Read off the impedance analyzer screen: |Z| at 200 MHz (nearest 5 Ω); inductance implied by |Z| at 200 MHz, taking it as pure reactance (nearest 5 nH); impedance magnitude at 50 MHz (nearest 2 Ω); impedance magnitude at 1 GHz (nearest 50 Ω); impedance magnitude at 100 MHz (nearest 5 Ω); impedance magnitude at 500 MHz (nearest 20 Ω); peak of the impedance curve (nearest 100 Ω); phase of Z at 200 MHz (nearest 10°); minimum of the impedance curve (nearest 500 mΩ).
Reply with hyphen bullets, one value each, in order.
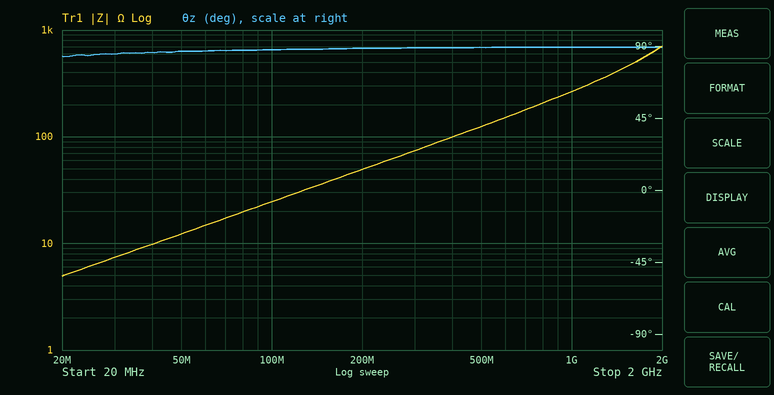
- 50 Ω
- 40 nH
- 12 Ω
- 250 Ω
- 25 Ω
- 120 Ω
- 700 Ω
- 90°
- 5.0 Ω
